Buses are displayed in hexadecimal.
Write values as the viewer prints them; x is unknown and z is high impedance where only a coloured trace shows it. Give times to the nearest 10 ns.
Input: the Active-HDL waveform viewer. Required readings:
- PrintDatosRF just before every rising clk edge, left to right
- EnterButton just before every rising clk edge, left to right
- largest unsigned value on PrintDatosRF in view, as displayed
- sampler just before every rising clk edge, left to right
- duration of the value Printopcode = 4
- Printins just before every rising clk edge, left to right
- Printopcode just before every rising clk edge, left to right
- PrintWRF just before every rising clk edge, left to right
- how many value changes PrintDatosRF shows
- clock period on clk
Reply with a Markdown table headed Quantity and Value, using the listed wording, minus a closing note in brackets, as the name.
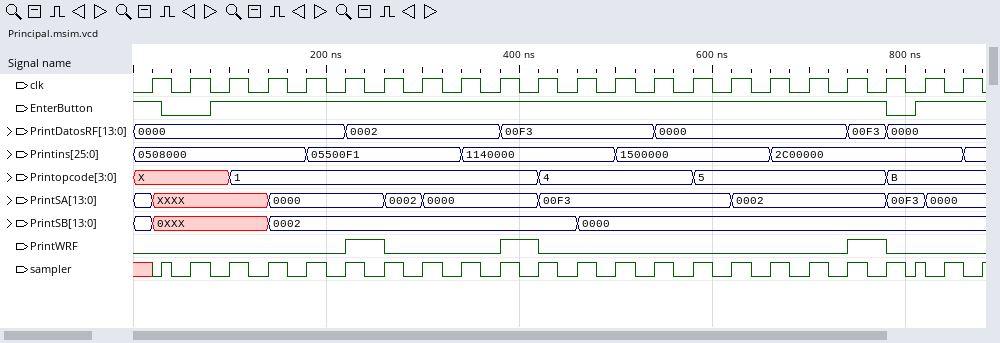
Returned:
| Quantity | Value |
|---|---|
| PrintDatosRF just before every rising clk edge, left to right | 0000, 0000, 0000, 0000, 0000, 0000, 0002, 0002, 0002, 0002, 00F3, 00F3, 00F3, 00F3, 0000, 0000, 0000, 0000, 0000, 00F3, 0000, 0000 |
| EnterButton just before every rising clk edge, left to right | 1 0 1 1 1 1 1 1 1 1 1 1 1 1 1 1 1 1 1 1 1 1 |
| largest unsigned value on PrintDatosRF in view, as displayed | 00F3 |
| sampler just before every rising clk edge, left to right | x 0 0 0 0 0 0 0 0 0 0 0 0 0 0 0 0 0 0 0 1 1 |
| duration of the value Printopcode = 4 | 160 ns |
| Printins just before every rising clk edge, left to right | 0508000, 0508000, 0508000, 0508000, 0508000, 05500F1, 05500F1, 05500F1, 05500F1, 1140000, 1140000, 1140000, 1140000, 1500000, 1500000, 1500000, 1500000, 2C00000, 2C00000, 2C00000, 2C00000, 2C00000 |
| Printopcode just before every rising clk edge, left to right | X, X, X, 1, 1, 1, 1, 1, 1, 1, 1, 4, 4, 4, 4, 5, 5, 5, 5, 5, B, B |
| PrintWRF just before every rising clk edge, left to right | 0 0 0 0 0 0 1 0 0 0 1 0 0 0 0 0 0 0 0 1 0 0 |
| how many value changes PrintDatosRF shows | 5 |
| clock period on clk | 40 ns |
